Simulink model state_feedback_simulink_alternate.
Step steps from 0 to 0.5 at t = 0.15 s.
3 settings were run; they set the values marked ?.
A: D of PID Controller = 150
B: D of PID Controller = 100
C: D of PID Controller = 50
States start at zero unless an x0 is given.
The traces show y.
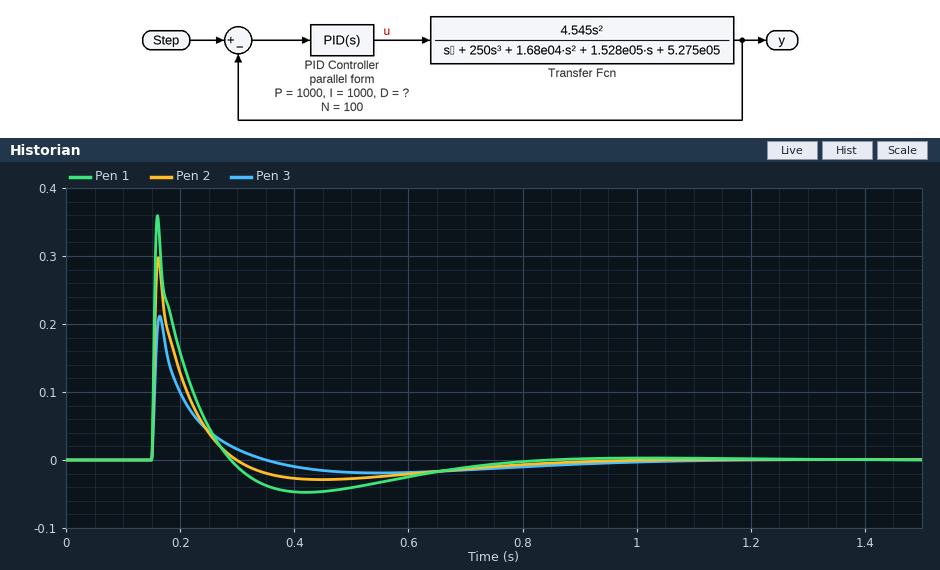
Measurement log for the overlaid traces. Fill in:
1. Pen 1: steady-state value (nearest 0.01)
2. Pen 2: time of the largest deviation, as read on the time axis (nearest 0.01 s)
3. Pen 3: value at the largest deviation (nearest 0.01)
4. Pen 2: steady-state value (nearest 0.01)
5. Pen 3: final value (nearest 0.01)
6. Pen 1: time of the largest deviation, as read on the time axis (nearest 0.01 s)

0.00
0.16 s
0.21
0.00
0.00
0.16 s
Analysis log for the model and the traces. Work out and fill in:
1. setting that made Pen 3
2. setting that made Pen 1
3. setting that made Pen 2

C
A
B
